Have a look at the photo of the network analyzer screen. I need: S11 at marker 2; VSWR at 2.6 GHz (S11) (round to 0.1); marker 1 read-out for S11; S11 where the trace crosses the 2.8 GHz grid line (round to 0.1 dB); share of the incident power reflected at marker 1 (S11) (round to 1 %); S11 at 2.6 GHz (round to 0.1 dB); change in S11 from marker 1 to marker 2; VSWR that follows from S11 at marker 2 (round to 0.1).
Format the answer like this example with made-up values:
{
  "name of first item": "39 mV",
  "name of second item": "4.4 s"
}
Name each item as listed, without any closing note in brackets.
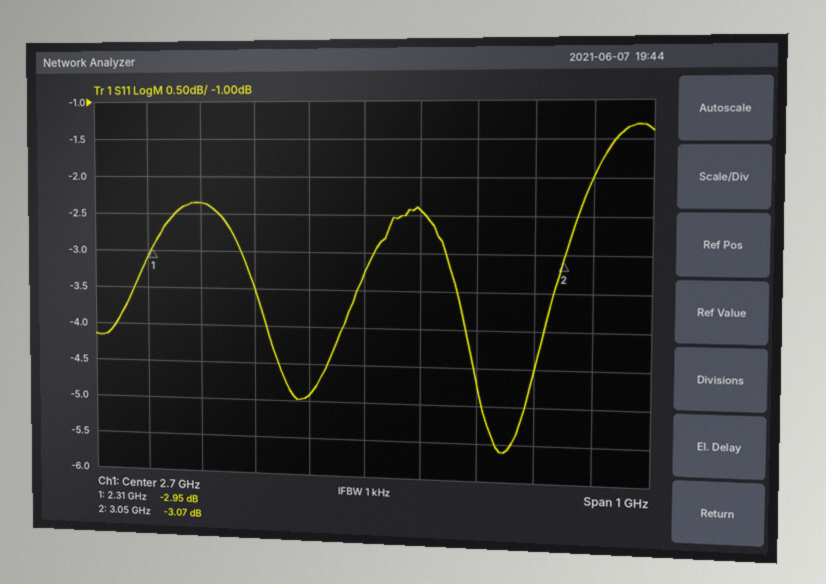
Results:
{
  "S11 at marker 2": "-3.07 dB",
  "VSWR at 2.6 GHz (S11)": "3.6",
  "marker 1 read-out for S11": "-2.95 dB",
  "S11 where the trace crosses the 2.8 GHz grid line": "-2.4 dB",
  "share of the incident power reflected at marker 1 (S11)": "51 %",
  "S11 at 2.6 GHz": "-4.9 dB",
  "change in S11 from marker 1 to marker 2": "-0.12 dB",
  "VSWR that follows from S11 at marker 2": "5.7"
}
